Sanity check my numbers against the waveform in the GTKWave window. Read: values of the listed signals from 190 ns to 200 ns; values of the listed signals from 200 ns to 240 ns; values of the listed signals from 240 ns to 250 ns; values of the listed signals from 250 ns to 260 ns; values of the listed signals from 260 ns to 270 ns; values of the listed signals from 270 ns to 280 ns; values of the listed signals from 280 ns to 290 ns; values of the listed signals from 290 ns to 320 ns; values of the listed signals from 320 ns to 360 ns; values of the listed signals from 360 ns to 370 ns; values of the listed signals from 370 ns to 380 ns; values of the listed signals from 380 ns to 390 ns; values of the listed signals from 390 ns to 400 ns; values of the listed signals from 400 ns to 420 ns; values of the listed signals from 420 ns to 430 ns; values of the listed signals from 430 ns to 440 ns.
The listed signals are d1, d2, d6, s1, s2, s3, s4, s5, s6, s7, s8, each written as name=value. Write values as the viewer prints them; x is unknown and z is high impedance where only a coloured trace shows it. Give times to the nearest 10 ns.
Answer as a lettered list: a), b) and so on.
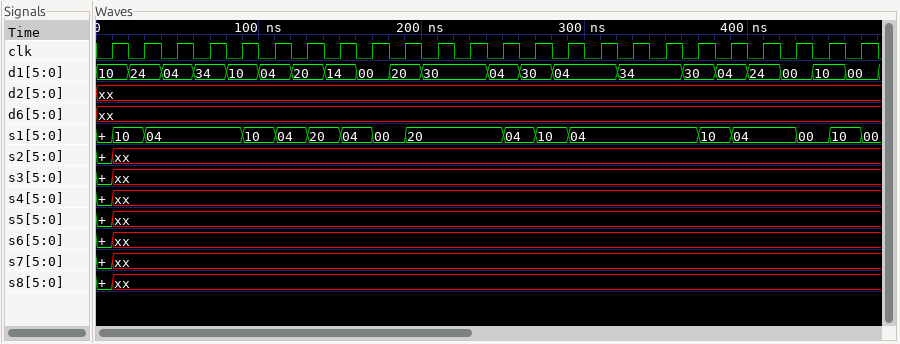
a) d1=20, d2=xx, d6=xx, s1=20, s2=xx, s3=xx, s4=xx, s5=xx, s6=xx, s7=xx, s8=xx
b) d1=30, d2=xx, d6=xx, s1=20, s2=xx, s3=xx, s4=xx, s5=xx, s6=xx, s7=xx, s8=xx
c) d1=04, d2=xx, d6=xx, s1=20, s2=xx, s3=xx, s4=xx, s5=xx, s6=xx, s7=xx, s8=xx
d) d1=04, d2=xx, d6=xx, s1=04, s2=xx, s3=xx, s4=xx, s5=xx, s6=xx, s7=xx, s8=xx
e) d1=30, d2=xx, d6=xx, s1=04, s2=xx, s3=xx, s4=xx, s5=xx, s6=xx, s7=xx, s8=xx
f) d1=30, d2=xx, d6=xx, s1=10, s2=xx, s3=xx, s4=xx, s5=xx, s6=xx, s7=xx, s8=xx
g) d1=04, d2=xx, d6=xx, s1=10, s2=xx, s3=xx, s4=xx, s5=xx, s6=xx, s7=xx, s8=xx
h) d1=04, d2=xx, d6=xx, s1=04, s2=xx, s3=xx, s4=xx, s5=xx, s6=xx, s7=xx, s8=xx
i) d1=34, d2=xx, d6=xx, s1=04, s2=xx, s3=xx, s4=xx, s5=xx, s6=xx, s7=xx, s8=xx
j) d1=30, d2=xx, d6=xx, s1=04, s2=xx, s3=xx, s4=xx, s5=xx, s6=xx, s7=xx, s8=xx
k) d1=30, d2=xx, d6=xx, s1=10, s2=xx, s3=xx, s4=xx, s5=xx, s6=xx, s7=xx, s8=xx
l) d1=04, d2=xx, d6=xx, s1=10, s2=xx, s3=xx, s4=xx, s5=xx, s6=xx, s7=xx, s8=xx
m) d1=04, d2=xx, d6=xx, s1=04, s2=xx, s3=xx, s4=xx, s5=xx, s6=xx, s7=xx, s8=xx
n) d1=24, d2=xx, d6=xx, s1=04, s2=xx, s3=xx, s4=xx, s5=xx, s6=xx, s7=xx, s8=xx
o) d1=00, d2=xx, d6=xx, s1=04, s2=xx, s3=xx, s4=xx, s5=xx, s6=xx, s7=xx, s8=xx
p) d1=00, d2=xx, d6=xx, s1=00, s2=xx, s3=xx, s4=xx, s5=xx, s6=xx, s7=xx, s8=xx
